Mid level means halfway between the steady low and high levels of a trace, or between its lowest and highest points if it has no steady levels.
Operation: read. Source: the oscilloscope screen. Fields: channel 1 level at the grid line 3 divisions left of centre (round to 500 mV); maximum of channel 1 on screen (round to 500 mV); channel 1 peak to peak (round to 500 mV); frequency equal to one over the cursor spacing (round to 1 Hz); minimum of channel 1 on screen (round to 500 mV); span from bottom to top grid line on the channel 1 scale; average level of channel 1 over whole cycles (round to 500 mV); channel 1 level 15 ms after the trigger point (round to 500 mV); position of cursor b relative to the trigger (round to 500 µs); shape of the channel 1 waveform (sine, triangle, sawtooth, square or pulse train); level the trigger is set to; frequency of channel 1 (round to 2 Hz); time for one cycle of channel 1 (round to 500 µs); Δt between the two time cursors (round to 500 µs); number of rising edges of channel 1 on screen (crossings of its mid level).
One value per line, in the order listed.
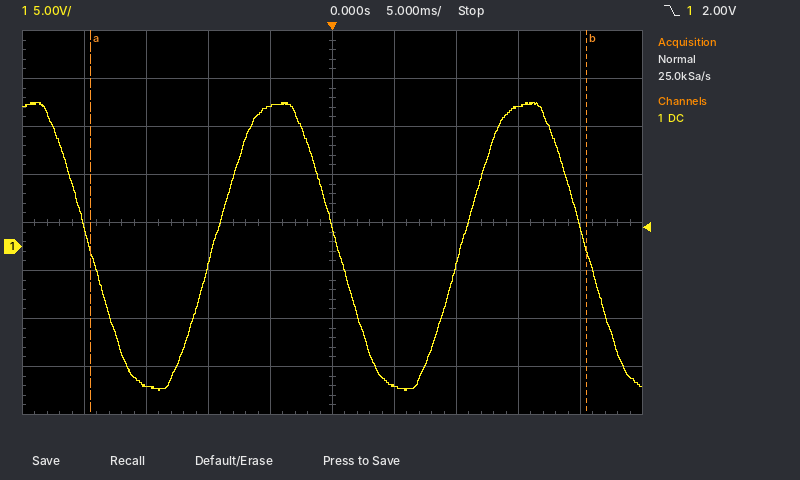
-14.5 V
15.0 V
30.0 V
25 Hz
-15.0 V
40 V
0.0 V
14.5 V
+20.5 ms
sine
2.00 V
50 Hz
20.0 ms
40.0 ms
2
